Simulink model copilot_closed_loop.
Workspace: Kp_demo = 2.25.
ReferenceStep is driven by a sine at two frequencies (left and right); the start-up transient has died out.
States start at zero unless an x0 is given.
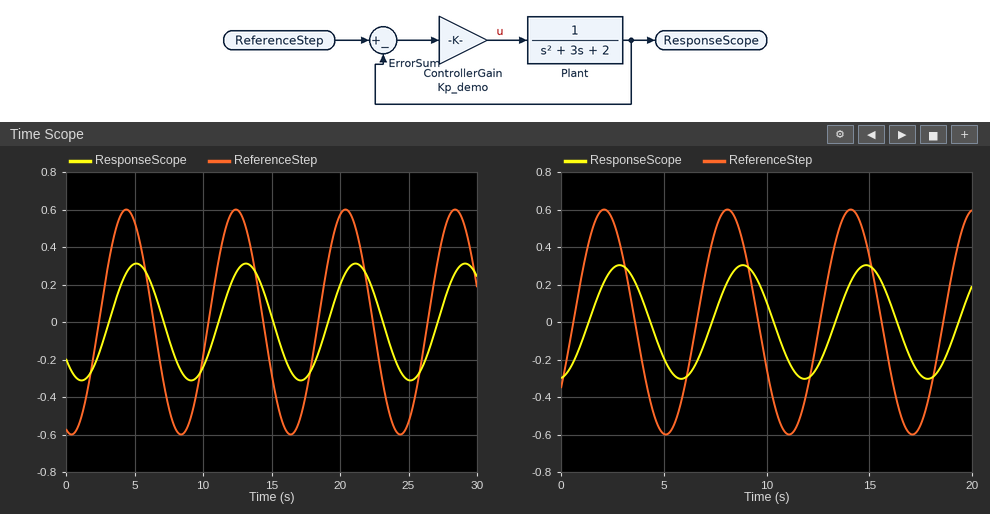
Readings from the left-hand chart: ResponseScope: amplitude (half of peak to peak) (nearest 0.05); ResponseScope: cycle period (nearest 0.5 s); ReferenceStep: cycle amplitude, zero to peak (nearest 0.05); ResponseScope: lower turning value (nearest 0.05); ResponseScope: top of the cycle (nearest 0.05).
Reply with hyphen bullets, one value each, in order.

- 0.30
- 8.0 s
- 0.60
- -0.30
- 0.30
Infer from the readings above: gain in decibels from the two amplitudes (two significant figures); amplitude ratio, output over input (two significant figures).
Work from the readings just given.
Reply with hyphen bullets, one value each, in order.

- -6.0 dB
- 0.50
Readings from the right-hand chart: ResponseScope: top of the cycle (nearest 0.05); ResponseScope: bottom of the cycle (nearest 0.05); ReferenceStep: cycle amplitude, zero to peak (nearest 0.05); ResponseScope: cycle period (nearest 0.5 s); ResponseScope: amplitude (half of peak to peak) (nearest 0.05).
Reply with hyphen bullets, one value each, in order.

- 0.30
- -0.30
- 0.60
- 6.0 s
- 0.30
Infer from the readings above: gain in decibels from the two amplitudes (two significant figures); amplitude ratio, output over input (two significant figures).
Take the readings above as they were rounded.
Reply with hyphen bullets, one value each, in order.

- -6.0 dB
- 0.50
